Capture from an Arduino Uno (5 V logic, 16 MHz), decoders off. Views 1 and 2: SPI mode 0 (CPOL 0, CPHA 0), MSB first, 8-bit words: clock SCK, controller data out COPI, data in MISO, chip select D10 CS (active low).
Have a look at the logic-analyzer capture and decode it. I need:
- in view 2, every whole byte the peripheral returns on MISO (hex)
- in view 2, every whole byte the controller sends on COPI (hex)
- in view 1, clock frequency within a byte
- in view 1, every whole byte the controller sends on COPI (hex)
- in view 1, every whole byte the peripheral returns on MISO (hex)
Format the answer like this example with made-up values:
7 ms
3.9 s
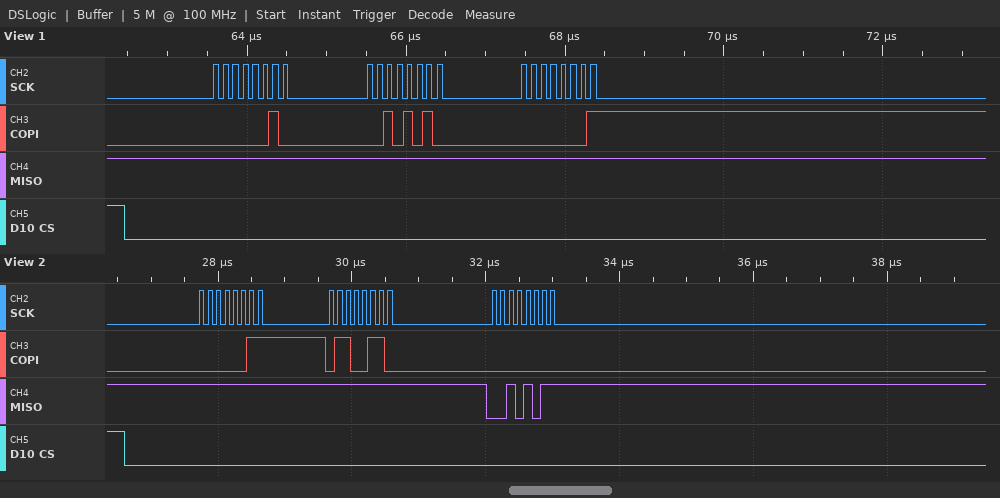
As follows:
0xFF 0xFF 0x2B
0x03 0x66 0x00
8 MHz
02 2A 01
FF FF FF
